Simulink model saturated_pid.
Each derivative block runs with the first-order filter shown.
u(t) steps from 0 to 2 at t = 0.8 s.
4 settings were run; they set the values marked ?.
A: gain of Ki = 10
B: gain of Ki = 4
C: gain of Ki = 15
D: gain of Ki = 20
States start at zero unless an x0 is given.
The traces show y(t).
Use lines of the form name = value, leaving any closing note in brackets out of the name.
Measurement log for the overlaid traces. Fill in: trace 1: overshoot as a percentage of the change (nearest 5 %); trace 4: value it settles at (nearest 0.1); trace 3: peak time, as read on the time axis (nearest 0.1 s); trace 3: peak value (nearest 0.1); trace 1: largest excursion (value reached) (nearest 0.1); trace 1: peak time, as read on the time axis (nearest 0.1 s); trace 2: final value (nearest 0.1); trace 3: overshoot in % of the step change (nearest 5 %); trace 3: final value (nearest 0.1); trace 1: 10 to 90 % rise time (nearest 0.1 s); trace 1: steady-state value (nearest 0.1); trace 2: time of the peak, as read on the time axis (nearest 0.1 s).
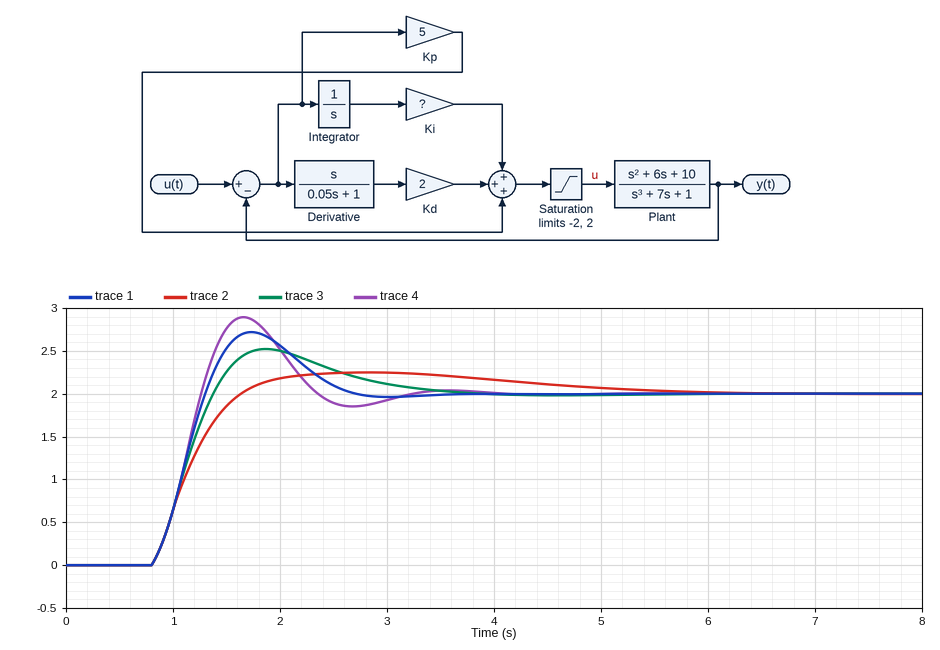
trace 1: overshoot as a percentage of the change = 35 %
trace 4: value it settles at = 2.0
trace 3: peak time, as read on the time axis = 1.9 s
trace 3: peak value = 2.5
trace 1: largest excursion (value reached) = 2.7
trace 1: peak time, as read on the time axis = 1.7 s
trace 2: final value = 2.0
trace 3: overshoot in % of the step change = 25 %
trace 3: final value = 2.0
trace 1: 10 to 90 % rise time = 0.4 s
trace 1: steady-state value = 2.0
trace 2: time of the peak, as read on the time axis = 2.8 s
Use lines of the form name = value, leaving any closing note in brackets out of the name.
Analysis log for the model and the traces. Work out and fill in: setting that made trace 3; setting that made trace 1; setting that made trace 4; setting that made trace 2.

setting that made trace 3 = A
setting that made trace 1 = C
setting that made trace 4 = D
setting that made trace 2 = B
